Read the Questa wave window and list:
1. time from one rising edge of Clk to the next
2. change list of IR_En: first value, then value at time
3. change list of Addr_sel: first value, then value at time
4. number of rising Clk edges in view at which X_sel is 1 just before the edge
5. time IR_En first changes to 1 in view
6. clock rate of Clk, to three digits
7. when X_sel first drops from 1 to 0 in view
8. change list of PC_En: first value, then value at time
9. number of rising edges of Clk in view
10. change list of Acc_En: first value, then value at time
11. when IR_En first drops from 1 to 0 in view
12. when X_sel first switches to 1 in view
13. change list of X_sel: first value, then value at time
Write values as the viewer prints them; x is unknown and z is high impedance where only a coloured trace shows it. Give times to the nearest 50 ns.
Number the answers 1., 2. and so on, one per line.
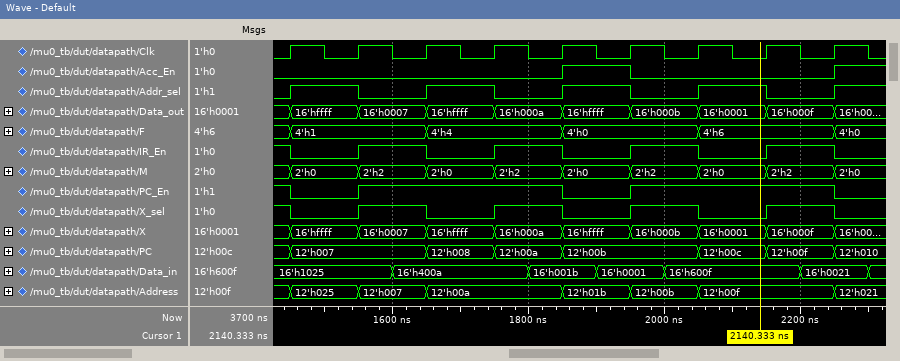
1. 100 ns
2. 1, 0 at 1450 ns, 1 at 1550 ns, 0 at 1650 ns, 1 at 1750 ns, 0 at 1850 ns, 1 at 1950 ns, 0 at 2050 ns, 1 at 2150 ns, 0 at 2250 ns
3. 0, 1 at 1450 ns, 0 at 1550 ns, 1 at 1650 ns, 0 at 1750 ns, 1 at 1850 ns, 0 at 1950 ns, 1 at 2050 ns, 0 at 2150 ns, 1 at 2250 ns
4. 5
5. 1550 ns
6. 10.0 MHz
7. 1450 ns
8. 1, 0 at 1450 ns, 1 at 1550 ns, 0 at 1850 ns, 1 at 1950 ns, 0 at 2250 ns
9. 9
10. 0, 1 at 1850 ns, 0 at 1950 ns, 1 at 2250 ns
11. 1450 ns
12. 1550 ns
13. 1, 0 at 1450 ns, 1 at 1550 ns, 0 at 1650 ns, 1 at 1750 ns, 0 at 1850 ns, 1 at 1950 ns, 0 at 2050 ns, 1 at 2150 ns, 0 at 2250 ns
